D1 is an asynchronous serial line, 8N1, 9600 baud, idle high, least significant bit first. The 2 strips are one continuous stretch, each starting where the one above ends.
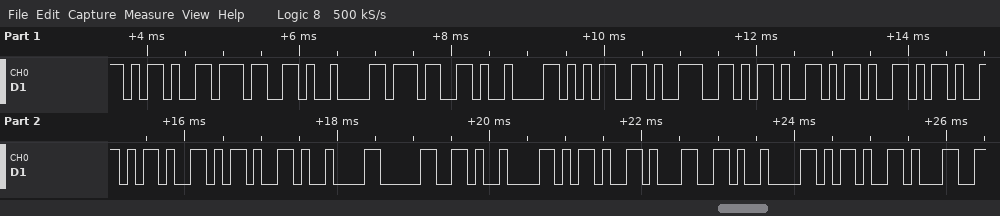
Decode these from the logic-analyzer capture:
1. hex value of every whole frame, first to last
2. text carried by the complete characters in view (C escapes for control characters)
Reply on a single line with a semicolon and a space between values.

2D 37 09 37 09 35 39 2D 2D 2D 2D 2D 09 30 09 2D 31 09 2D 31; "-7\t7\t59-----\t0\t-1\t-1"
